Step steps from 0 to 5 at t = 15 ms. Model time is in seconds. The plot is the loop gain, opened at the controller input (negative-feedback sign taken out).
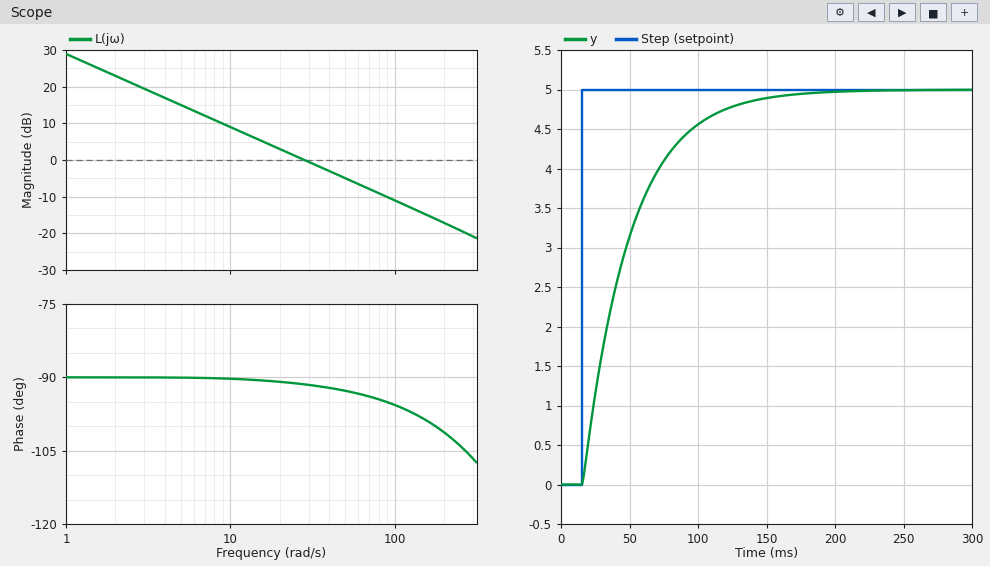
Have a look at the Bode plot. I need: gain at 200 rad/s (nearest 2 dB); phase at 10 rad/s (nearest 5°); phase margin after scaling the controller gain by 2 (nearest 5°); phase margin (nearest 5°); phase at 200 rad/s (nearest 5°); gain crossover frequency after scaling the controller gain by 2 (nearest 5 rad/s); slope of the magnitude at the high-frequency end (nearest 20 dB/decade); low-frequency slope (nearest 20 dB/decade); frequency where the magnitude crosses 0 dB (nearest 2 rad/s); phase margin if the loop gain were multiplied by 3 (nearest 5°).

-18 dB
-90°
85°
90°
-100°
55 rad/s
-20 dB/decade
-20 dB/decade
28 rad/s
85°
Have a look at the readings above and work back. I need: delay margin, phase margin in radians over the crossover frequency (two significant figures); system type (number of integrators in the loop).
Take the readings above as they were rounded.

0.056 s
1
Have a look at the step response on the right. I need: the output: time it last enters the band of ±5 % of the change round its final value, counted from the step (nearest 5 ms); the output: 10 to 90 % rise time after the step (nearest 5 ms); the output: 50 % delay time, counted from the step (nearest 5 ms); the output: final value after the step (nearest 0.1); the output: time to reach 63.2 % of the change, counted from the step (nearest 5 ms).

105 ms
75 ms
25 ms
5.0
35 ms
